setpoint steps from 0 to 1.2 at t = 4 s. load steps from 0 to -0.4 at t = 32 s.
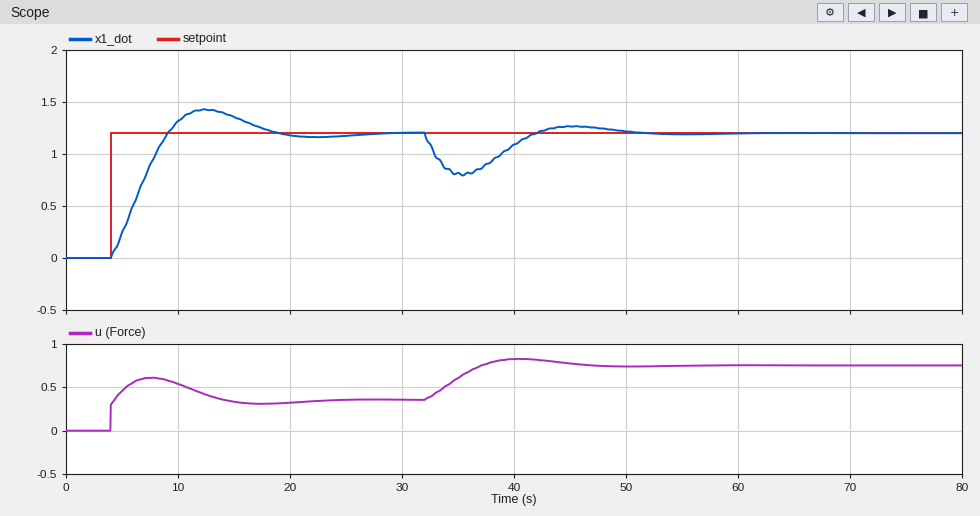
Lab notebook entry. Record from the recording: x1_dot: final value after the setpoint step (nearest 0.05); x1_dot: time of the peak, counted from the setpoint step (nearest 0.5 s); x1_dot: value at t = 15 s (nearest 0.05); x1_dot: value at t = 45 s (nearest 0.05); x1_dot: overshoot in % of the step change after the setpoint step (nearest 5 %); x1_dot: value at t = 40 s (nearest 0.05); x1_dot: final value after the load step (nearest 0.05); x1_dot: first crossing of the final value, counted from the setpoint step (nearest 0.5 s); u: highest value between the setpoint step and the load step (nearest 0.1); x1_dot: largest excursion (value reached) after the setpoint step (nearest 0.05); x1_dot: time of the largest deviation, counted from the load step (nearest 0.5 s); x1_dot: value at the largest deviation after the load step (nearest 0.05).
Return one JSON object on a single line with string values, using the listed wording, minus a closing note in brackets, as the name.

{"x1_dot: final value after the setpoint step": "1.20", "x1_dot: time of the peak, counted from the setpoint step": "8.5 s", "x1_dot: value at t = 15 s": "1.35", "x1_dot: value at t = 45 s": "1.25", "x1_dot: overshoot in % of the step change after the setpoint step": "20 %", "x1_dot: value at t = 40 s": "1.10", "x1_dot: final value after the load step": "1.20", "x1_dot: first crossing of the final value, counted from the setpoint step": "5.0 s", "u: highest value between the setpoint step and the load step": "0.6", "x1_dot: largest excursion (value reached) after the setpoint step": "1.45", "x1_dot: time of the largest deviation, counted from the load step": "3.5 s", "x1_dot: value at the largest deviation after the load step": "0.80"}
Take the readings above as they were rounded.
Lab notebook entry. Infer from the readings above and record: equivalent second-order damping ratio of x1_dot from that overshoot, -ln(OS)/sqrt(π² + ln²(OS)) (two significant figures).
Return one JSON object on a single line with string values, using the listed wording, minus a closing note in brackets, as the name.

{"equivalent second-order damping ratio of x1_dot from that overshoot, -ln(OS)/sqrt(π² + ln²(OS))": "0.46"}
